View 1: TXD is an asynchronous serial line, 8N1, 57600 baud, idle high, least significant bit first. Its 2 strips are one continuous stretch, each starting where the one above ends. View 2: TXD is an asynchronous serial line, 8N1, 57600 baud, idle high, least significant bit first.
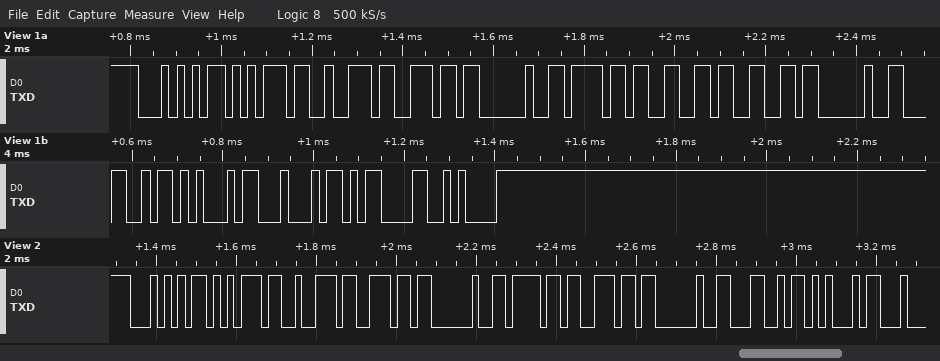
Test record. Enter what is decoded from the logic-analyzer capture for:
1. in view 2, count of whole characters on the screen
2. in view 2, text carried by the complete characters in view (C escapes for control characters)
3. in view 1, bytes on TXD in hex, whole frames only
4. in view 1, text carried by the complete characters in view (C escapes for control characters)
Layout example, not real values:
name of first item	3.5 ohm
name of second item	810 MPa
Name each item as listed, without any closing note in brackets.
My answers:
in view 2, count of whole characters on the screen	10
in view 2, text carried by the complete characters in view	"Turn on LE"
in view 1, bytes on TXD in hex, whole frames only	54 75 72 6E 20 6F 66 66 20 4C 45 44 0D 0A
in view 1, text carried by the complete characters in view	"Turn off LED\r\n"
